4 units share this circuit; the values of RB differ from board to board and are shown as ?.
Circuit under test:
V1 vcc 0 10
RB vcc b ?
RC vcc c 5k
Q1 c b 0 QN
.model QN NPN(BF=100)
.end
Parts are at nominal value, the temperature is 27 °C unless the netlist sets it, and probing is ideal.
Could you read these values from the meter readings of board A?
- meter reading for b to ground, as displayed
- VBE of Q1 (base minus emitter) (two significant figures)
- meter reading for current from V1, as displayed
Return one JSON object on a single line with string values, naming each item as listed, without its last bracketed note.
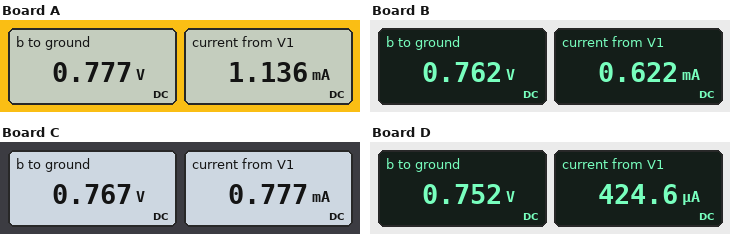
{"meter reading for b to ground, as displayed": "0.777 V", "VBE of Q1 (base minus emitter)": "780 mV", "meter reading for current from V1, as displayed": "1.136 mA"}
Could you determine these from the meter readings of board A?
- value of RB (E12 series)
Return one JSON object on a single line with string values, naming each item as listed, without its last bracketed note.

{"value of RB": "820 kΩ"}
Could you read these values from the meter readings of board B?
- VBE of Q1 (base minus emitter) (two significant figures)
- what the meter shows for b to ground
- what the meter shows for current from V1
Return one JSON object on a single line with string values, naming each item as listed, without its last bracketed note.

{"VBE of Q1 (base minus emitter)": "760 mV", "what the meter shows for b to ground": "0.762 V", "what the meter shows for current from V1": "0.622 mA"}
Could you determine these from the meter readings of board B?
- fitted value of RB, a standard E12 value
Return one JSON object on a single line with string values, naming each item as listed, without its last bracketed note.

{"fitted value of RB, a standard E12 value": "1.5 MΩ"}
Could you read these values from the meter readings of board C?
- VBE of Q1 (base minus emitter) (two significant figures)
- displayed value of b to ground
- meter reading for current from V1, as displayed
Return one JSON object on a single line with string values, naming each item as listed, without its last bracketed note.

{"VBE of Q1 (base minus emitter)": "770 mV", "displayed value of b to ground": "0.767 V", "meter reading for current from V1, as displayed": "0.777 mA"}
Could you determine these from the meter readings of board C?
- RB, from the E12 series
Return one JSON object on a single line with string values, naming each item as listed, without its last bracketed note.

{"RB, from the E12 series": "1.2 MΩ"}
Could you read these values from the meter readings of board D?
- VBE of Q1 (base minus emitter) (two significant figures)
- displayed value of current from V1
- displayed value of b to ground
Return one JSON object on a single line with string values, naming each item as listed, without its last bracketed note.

{"VBE of Q1 (base minus emitter)": "750 mV", "displayed value of current from V1": "424.6 µA", "displayed value of b to ground": "0.752 V"}
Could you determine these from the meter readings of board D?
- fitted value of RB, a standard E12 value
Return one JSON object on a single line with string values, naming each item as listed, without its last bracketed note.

{"fitted value of RB, a standard E12 value": "2.2 MΩ"}
